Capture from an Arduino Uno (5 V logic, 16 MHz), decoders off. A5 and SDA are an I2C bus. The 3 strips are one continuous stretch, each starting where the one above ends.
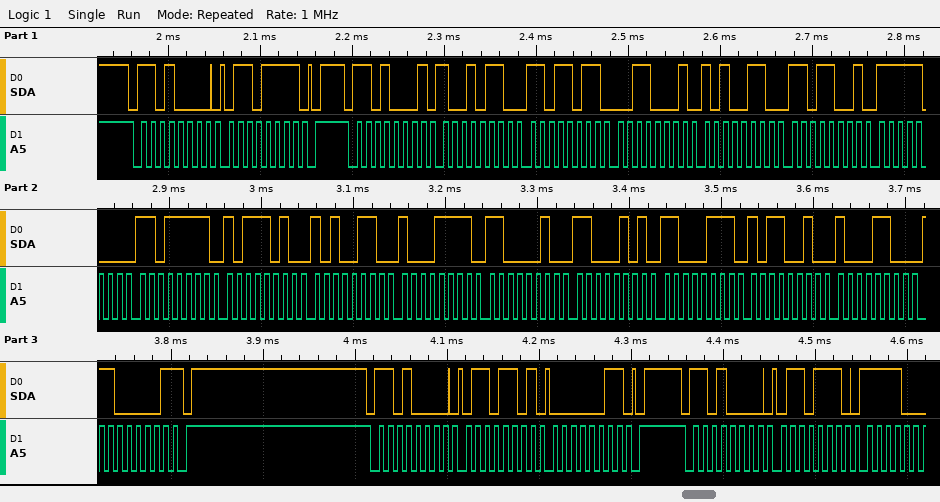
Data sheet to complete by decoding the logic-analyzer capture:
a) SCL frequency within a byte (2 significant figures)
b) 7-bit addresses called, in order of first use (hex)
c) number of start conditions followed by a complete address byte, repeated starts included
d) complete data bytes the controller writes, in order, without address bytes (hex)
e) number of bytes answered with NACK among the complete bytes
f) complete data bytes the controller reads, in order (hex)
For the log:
100 kHz
0x68
4
6F 6D 03 6E
1
96 DB 31 A6 D9 F8 DF BA A6 8F C2 C5 C7 B2 8C C1
